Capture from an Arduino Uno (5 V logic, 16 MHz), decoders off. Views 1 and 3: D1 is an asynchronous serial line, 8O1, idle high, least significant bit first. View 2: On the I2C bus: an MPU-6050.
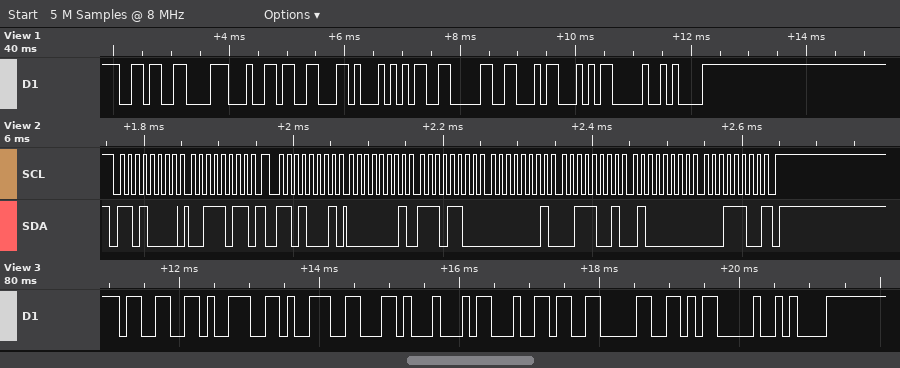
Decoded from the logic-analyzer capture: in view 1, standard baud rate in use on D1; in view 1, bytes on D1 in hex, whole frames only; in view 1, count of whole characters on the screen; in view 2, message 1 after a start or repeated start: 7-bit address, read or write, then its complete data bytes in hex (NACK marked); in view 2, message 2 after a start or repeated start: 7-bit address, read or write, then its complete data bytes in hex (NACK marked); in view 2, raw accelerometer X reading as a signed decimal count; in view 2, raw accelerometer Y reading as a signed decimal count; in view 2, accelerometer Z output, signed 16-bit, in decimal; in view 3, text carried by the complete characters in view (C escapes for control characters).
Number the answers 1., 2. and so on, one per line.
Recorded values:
1. 9600 baud
2. 36 38 36 2C 35 30 34 0D 0A
3. 9
4. 0x68 write: 3B
5. 0x68 read: 01 EC 01 39 40 1C NACK
6. 492
7. 313
8. 16412
9. "399,460\r\n"
